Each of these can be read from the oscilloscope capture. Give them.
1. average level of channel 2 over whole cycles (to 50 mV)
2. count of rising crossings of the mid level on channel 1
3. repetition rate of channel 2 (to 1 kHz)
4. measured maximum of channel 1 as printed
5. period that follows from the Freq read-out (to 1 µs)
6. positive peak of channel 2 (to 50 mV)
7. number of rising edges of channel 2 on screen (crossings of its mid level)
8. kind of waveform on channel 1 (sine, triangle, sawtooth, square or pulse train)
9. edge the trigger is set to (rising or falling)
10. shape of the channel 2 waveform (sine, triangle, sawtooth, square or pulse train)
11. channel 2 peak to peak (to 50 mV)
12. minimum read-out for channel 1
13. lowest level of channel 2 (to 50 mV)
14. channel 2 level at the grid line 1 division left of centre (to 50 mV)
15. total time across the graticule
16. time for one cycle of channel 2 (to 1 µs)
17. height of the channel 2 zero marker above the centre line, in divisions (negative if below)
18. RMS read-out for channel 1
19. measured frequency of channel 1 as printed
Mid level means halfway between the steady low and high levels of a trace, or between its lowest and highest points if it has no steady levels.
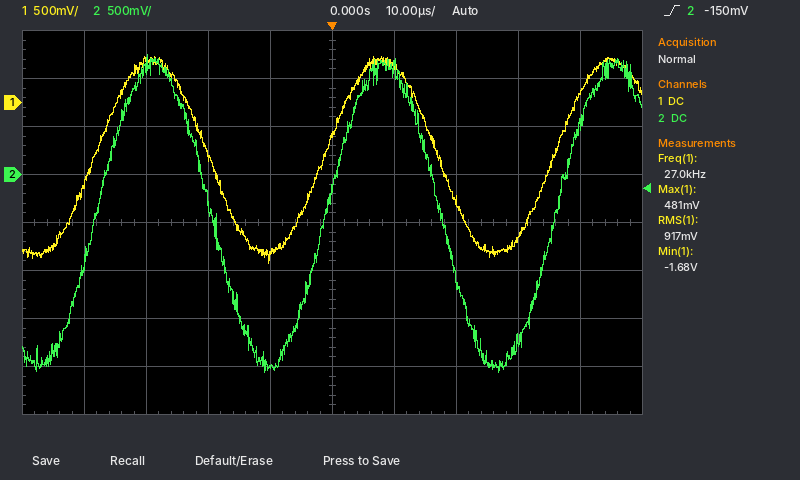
-400 mV
3
27 kHz
481 mV
37 µs
1.25 V
3
sine
rising
sine
3.30 V
-1.68 V
-2.05 V
-2.00 V
100 µs
37 µs
+1.0 div
917 mV
27.0 kHz
